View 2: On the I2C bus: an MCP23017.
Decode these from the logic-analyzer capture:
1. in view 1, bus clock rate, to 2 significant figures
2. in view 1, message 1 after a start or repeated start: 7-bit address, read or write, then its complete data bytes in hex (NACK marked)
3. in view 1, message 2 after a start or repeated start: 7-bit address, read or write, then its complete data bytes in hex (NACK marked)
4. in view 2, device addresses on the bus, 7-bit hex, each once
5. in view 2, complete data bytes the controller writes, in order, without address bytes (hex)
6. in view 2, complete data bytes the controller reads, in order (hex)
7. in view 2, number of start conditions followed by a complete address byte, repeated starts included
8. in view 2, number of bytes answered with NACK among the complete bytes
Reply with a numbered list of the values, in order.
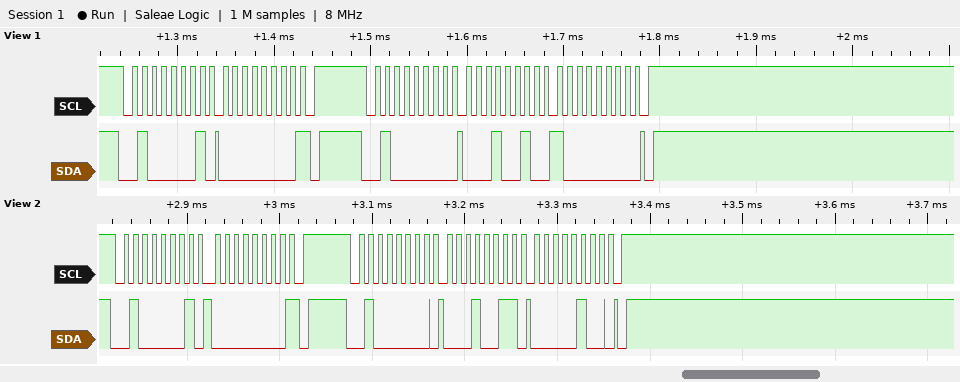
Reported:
1. 100 kHz
2. 0x20 read: 00 NACK
3. 0x20 write: 12 80
4. 0x20
5. 13 04
6. 00
7. 2
8. 1
